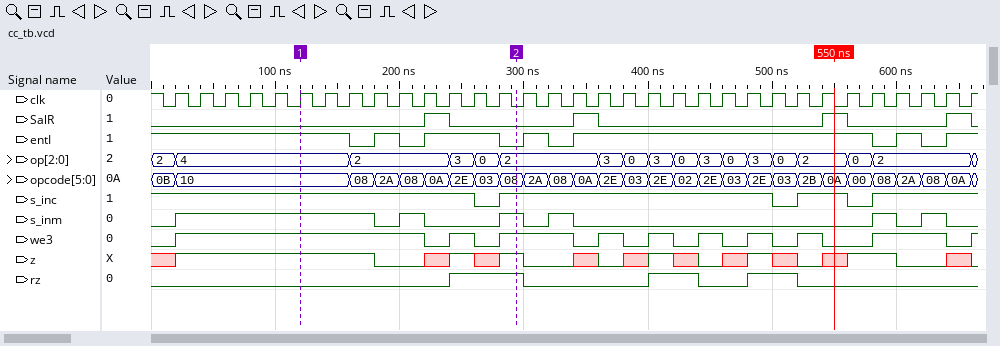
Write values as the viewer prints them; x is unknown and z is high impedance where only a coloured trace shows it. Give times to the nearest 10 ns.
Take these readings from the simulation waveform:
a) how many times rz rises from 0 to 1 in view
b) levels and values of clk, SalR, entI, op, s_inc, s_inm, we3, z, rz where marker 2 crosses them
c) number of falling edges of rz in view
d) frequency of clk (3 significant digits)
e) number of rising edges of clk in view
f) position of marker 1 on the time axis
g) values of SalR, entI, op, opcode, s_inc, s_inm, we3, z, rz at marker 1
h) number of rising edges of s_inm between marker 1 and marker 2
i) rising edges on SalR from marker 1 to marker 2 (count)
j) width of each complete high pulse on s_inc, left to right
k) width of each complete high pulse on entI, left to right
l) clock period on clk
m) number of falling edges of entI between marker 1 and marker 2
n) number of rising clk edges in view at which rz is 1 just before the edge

3
clk=0, SalR=0, entI=0, op=2, s_inc=1, s_inm=1, we3=1, z=1, rz=1
3
50.0 MHz
33
120 ns
SalR=0, entI=1, op=4, opcode=10, s_inc=1, s_inm=1, we3=1, z=1, rz=0
2
1
220 ns, 40 ns
20 ns, 60 ns, 20 ns, 240 ns, 20 ns
20 ns
3
7
